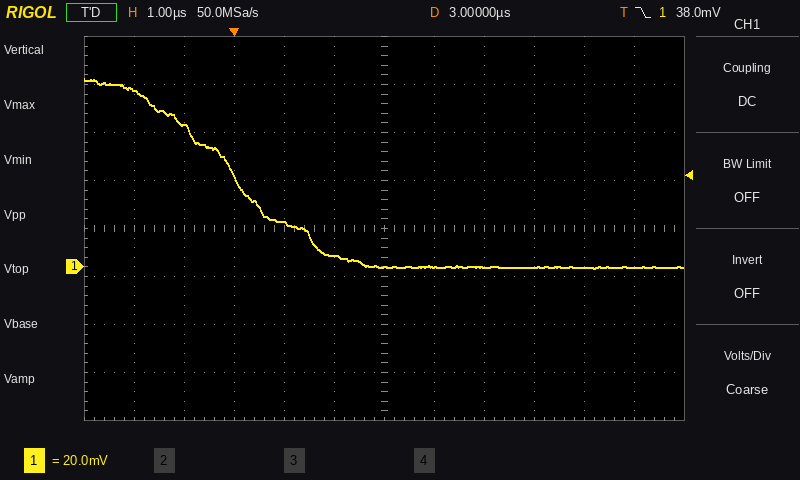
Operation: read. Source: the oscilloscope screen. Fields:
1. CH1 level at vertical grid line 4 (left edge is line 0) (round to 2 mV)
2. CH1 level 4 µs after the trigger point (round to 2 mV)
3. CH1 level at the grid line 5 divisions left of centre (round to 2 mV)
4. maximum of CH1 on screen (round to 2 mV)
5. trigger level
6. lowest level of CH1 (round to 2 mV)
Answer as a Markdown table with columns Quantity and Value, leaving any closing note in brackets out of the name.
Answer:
| Quantity | Value |
|---|---|
| CH1 level at vertical grid line 4 (left edge is line 0) | 18 mV |
| CH1 level 4 µs after the trigger point | 0 mV |
| CH1 level at the grid line 5 divisions left of centre | 74 mV |
| maximum of CH1 on screen | 78 mV |
| trigger level | 38.0 mV |
| lowest level of CH1 | 0 mV |
